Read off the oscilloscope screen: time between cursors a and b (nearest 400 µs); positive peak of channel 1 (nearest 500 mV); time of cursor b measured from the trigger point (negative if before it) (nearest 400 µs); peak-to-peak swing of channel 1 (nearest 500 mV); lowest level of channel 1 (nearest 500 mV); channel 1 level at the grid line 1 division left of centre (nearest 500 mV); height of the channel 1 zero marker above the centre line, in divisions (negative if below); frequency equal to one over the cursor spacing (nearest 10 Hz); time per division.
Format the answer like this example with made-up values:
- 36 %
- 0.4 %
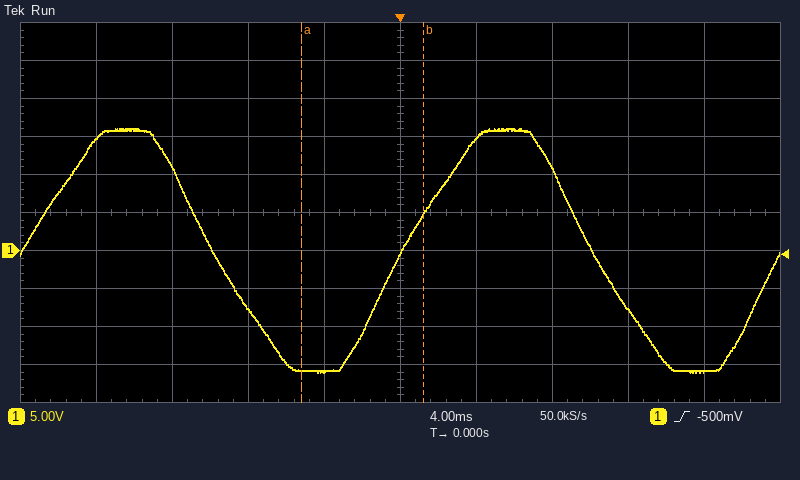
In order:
- 6.4 ms
- 16.0 V
- +1.2 ms
- 32.0 V
- -16.0 V
- -16.0 V
- -1.0 div
- 160 Hz
- 4 ms
